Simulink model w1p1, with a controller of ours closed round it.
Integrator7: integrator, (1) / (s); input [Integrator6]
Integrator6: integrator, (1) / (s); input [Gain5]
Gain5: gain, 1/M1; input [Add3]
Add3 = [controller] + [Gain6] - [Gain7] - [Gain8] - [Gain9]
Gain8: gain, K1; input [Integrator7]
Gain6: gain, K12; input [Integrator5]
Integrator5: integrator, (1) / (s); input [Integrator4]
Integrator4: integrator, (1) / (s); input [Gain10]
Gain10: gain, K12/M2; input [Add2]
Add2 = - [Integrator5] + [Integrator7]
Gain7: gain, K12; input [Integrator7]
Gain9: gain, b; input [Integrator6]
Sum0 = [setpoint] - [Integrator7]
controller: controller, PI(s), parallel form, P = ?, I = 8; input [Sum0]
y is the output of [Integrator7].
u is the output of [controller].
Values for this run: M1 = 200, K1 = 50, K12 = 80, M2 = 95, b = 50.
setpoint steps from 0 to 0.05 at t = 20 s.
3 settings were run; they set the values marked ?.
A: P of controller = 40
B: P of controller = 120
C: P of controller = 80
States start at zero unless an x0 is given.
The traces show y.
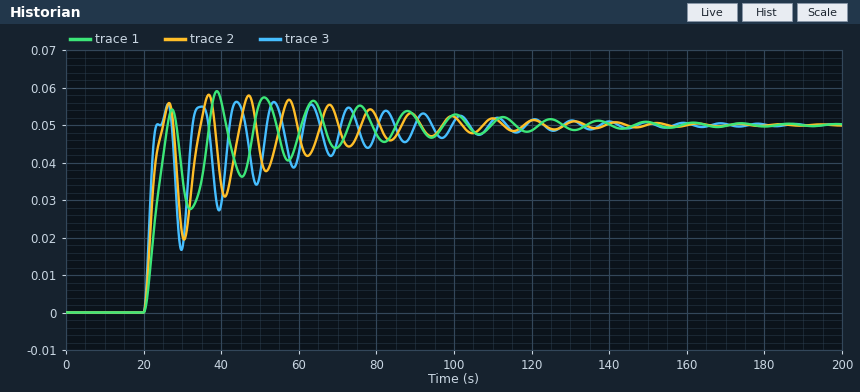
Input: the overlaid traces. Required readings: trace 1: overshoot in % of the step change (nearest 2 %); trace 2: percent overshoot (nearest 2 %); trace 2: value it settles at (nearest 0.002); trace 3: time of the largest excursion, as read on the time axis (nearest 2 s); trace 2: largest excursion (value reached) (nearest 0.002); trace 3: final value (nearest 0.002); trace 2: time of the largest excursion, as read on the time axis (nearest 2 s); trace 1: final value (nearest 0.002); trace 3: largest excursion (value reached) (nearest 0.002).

18 %
16 %
0.050
44 s
0.058
0.050
36 s
0.050
0.056
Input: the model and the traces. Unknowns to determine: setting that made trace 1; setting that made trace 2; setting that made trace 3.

A
C
B
